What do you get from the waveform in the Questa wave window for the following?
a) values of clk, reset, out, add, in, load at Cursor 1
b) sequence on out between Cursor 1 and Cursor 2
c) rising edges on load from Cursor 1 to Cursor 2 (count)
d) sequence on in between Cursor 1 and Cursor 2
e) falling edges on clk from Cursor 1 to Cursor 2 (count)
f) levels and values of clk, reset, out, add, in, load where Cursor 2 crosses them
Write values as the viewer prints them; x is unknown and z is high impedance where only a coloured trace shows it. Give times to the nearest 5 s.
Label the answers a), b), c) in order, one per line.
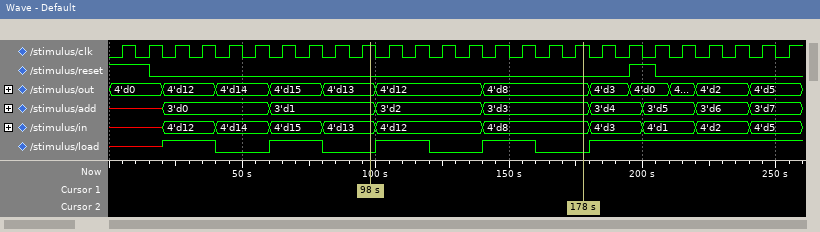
a) clk=1, reset=0, out=4'd13, add=3'd1, in=4'd13, load=0
b) 4'd13, 4'd12, 4'd8
c) 2
d) 4'd13, 4'd12, 4'd8
e) 8
f) clk=1, reset=0, out=4'd8, add=3'd3, in=4'd8, load=0
